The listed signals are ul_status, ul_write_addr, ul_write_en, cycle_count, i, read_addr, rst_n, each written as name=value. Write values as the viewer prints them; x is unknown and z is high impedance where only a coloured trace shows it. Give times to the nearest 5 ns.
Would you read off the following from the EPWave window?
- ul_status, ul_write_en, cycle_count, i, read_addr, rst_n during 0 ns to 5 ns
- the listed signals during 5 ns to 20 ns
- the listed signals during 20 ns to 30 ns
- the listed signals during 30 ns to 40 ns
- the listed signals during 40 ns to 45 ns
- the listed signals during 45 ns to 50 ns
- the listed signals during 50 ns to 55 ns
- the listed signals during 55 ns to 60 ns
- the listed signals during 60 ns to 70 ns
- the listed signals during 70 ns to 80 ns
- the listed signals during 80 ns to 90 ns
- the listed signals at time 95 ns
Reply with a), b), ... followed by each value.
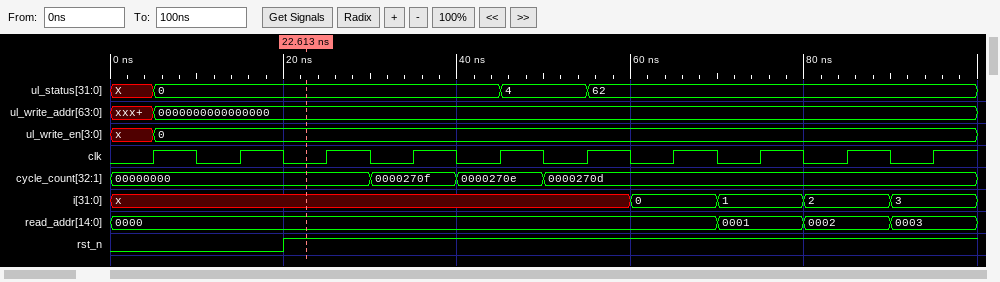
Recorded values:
a) ul_status=X, ul_write_en=x, cycle_count=00000000, i=x, read_addr=0000, rst_n=0
b) ul_status=0, ul_write_addr=0000000000000000, ul_write_en=0, cycle_count=00000000, i=x, read_addr=0000, rst_n=0
c) ul_status=0, ul_write_addr=0000000000000000, ul_write_en=0, cycle_count=00000000, i=x, read_addr=0000, rst_n=1
d) ul_status=0, ul_write_addr=0000000000000000, ul_write_en=0, cycle_count=0000270f, i=x, read_addr=0000, rst_n=1
e) ul_status=0, ul_write_addr=0000000000000000, ul_write_en=0, cycle_count=0000270e, i=x, read_addr=0000, rst_n=1
f) ul_status=4, ul_write_addr=0000000000000000, ul_write_en=0, cycle_count=0000270e, i=x, read_addr=0000, rst_n=1
g) ul_status=4, ul_write_addr=0000000000000000, ul_write_en=0, cycle_count=0000270d, i=x, read_addr=0000, rst_n=1
h) ul_status=62, ul_write_addr=0000000000000000, ul_write_en=0, cycle_count=0000270d, i=x, read_addr=0000, rst_n=1
i) ul_status=62, ul_write_addr=0000000000000000, ul_write_en=0, cycle_count=0000270d, i=0, read_addr=0000, rst_n=1
j) ul_status=62, ul_write_addr=0000000000000000, ul_write_en=0, cycle_count=0000270d, i=1, read_addr=0001, rst_n=1
k) ul_status=62, ul_write_addr=0000000000000000, ul_write_en=0, cycle_count=0000270d, i=2, read_addr=0002, rst_n=1
l) ul_status=62, ul_write_addr=0000000000000000, ul_write_en=0, cycle_count=0000270d, i=3, read_addr=0003, rst_n=1
